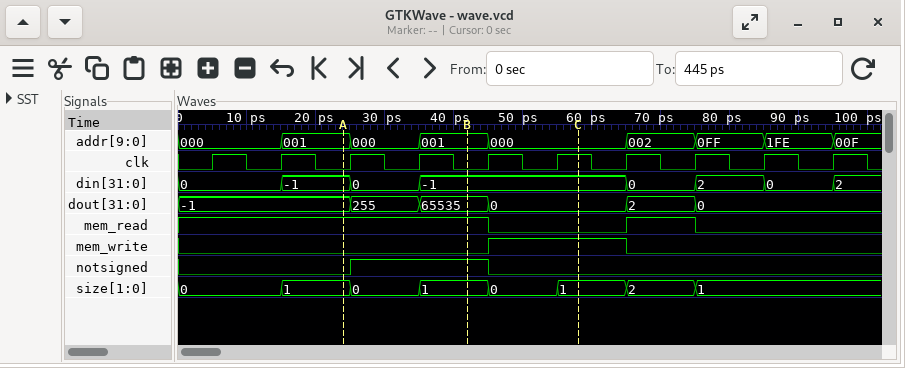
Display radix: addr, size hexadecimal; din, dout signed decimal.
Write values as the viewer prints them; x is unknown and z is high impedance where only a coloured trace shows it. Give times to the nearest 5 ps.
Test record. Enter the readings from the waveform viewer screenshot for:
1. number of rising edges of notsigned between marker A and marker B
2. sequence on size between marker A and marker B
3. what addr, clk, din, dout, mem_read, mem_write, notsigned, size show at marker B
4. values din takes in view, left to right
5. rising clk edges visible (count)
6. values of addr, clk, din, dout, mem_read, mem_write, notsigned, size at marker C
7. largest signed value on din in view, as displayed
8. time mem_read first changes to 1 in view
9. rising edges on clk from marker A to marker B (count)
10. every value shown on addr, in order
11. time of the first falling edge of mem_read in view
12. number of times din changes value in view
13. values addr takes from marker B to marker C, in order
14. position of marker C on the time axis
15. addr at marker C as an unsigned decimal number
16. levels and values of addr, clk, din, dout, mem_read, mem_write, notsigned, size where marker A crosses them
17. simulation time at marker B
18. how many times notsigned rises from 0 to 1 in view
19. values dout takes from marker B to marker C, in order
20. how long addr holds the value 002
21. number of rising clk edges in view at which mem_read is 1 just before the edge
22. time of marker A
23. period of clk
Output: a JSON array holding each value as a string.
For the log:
["1", "1, 0, 1", "addr=001, clk=0, din=-1, dout=65535, mem_read=1, mem_write=0, notsigned=1, size=1", "0, -1, 0, -1, 0, 2, 0, 2", "10", "addr=000, clk=1, din=-1, dout=0, mem_read=0, mem_write=1, notsigned=0, size=1", "2", "65 ps", "2", "000, 001, 000, 001, 000, 002, 0FF, 1FE, 00F", "45 ps", "7", "001, 000", "60 ps", "0", "addr=001, clk=0, din=-1, dout=-1, mem_read=1, mem_write=0, notsigned=0, size=1", "40 ps", "1", "65535, 0", "10 ps", "6", "25 ps", "10 ps"]
